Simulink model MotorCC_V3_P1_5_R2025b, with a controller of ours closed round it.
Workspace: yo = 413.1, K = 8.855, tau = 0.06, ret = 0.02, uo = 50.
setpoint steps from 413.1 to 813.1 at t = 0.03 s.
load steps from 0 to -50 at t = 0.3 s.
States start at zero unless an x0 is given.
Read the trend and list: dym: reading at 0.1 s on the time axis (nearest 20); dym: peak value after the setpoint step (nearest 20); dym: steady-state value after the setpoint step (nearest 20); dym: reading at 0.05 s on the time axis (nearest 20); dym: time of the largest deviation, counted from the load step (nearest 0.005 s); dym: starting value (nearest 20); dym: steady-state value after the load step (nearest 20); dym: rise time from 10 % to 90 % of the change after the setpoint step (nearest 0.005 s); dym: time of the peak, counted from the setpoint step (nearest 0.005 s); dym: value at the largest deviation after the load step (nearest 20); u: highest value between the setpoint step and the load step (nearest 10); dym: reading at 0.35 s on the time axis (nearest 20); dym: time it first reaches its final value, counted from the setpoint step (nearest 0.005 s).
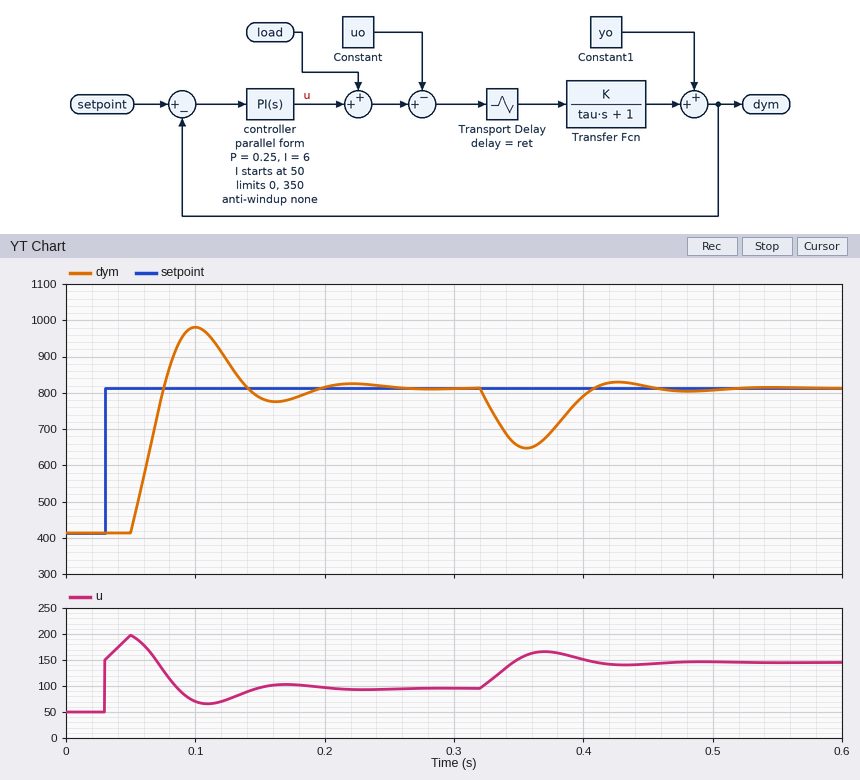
980
980
820
420
0.055 s
420
820
0.020 s
0.070 s
640
200
660
0.045 s
